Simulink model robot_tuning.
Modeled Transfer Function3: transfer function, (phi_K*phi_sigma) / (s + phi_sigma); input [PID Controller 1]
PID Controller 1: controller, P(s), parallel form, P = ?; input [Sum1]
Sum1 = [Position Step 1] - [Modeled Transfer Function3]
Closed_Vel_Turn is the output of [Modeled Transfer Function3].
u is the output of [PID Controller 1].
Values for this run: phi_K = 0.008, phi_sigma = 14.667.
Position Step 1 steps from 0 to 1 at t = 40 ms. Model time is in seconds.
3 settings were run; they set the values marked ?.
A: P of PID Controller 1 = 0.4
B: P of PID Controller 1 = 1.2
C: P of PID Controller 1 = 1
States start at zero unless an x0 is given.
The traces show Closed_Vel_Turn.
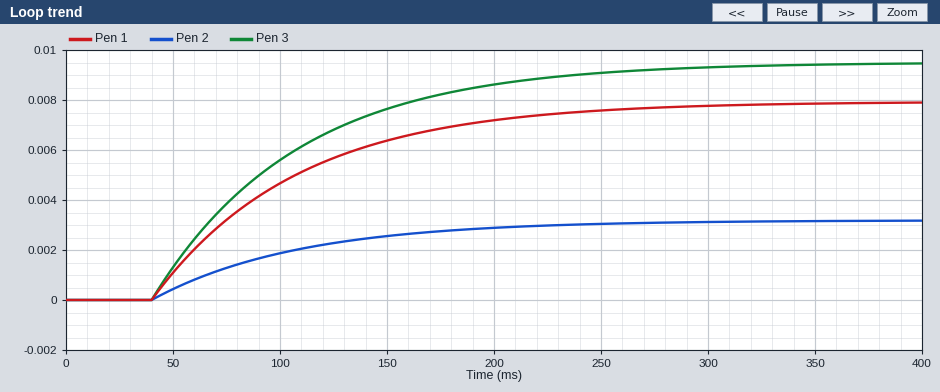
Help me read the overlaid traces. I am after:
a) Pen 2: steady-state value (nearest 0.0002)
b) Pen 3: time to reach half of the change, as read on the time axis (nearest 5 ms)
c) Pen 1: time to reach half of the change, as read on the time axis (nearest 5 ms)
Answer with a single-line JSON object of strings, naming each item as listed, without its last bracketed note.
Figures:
{"Pen 2: steady-state value": "0.0032", "Pen 3: time to reach half of the change, as read on the time axis": "85 ms", "Pen 1: time to reach half of the change, as read on the time axis": "85 ms"}
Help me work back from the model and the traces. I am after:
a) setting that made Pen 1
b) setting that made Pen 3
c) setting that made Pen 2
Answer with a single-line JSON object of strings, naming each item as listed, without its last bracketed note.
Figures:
{"setting that made Pen 1": "C", "setting that made Pen 3": "B", "setting that made Pen 2": "A"}
